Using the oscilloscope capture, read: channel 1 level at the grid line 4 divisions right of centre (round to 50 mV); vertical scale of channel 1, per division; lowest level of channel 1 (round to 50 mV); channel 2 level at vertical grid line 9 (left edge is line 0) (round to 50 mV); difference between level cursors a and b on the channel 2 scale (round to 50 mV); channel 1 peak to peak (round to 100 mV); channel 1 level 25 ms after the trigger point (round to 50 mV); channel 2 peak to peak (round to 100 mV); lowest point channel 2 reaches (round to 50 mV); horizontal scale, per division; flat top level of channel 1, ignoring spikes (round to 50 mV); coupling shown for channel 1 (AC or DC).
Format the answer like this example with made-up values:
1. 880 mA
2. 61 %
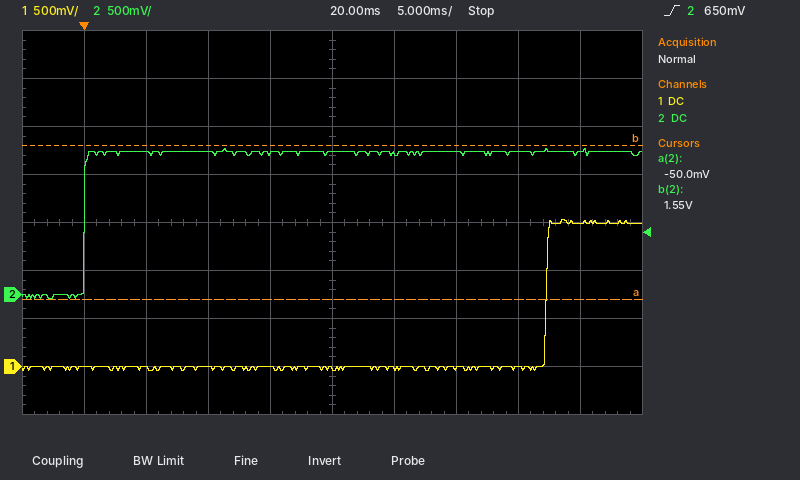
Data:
1. 1.50 V
2. 500 mV
3. -50 mV
4. 1.50 V
5. 1.60 V
6. 1.60 V
7. 0 mV
8. 1.60 V
9. -50 mV
10. 5 ms
11. 1.50 V
12. DC
